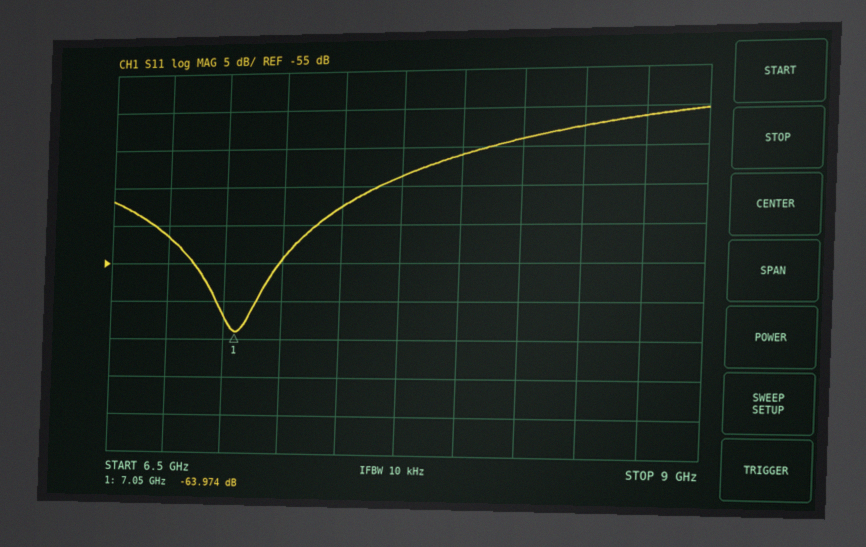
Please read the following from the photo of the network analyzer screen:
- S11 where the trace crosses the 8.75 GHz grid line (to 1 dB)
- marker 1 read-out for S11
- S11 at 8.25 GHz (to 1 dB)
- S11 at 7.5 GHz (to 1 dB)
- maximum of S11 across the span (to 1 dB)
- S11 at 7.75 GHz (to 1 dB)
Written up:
-36 dB
-63.974 dB
-39 dB
-48 dB
-35 dB
-44 dB
